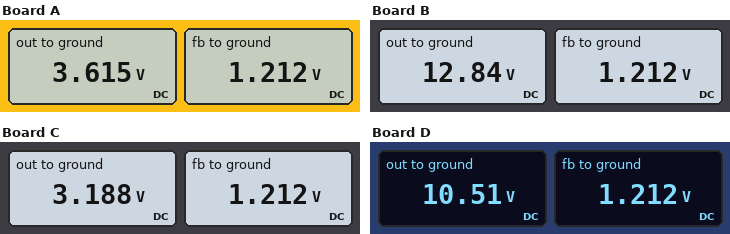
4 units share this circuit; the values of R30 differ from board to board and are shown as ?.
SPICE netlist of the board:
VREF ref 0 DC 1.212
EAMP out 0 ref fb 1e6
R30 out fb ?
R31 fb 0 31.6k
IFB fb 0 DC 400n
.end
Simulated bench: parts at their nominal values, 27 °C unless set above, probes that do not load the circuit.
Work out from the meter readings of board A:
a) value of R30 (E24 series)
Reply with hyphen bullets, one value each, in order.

- 62 kΩ
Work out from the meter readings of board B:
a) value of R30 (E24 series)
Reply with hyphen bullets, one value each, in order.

- 300 kΩ
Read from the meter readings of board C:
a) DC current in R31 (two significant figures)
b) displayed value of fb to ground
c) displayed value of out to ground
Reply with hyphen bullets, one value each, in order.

- 38 µA
- 1.212 V
- 3.188 V
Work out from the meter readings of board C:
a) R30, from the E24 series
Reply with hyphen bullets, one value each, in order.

- 51 kΩ
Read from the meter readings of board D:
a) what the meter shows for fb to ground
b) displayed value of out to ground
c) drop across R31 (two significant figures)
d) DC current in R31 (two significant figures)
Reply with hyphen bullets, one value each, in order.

- 1.212 V
- 10.51 V
- 1.2 V
- 38 µA
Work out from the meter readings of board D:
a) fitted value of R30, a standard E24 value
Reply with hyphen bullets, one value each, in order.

- 240 kΩ
